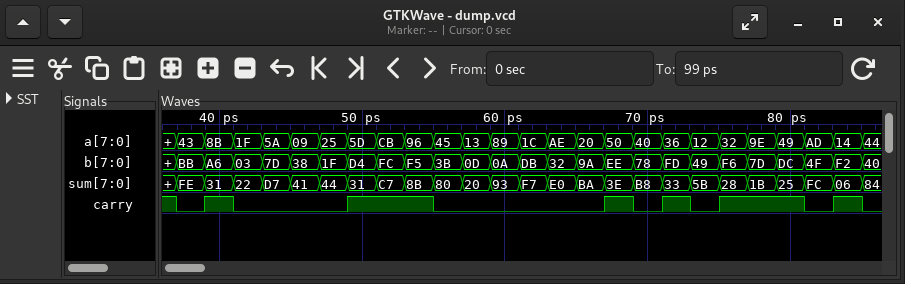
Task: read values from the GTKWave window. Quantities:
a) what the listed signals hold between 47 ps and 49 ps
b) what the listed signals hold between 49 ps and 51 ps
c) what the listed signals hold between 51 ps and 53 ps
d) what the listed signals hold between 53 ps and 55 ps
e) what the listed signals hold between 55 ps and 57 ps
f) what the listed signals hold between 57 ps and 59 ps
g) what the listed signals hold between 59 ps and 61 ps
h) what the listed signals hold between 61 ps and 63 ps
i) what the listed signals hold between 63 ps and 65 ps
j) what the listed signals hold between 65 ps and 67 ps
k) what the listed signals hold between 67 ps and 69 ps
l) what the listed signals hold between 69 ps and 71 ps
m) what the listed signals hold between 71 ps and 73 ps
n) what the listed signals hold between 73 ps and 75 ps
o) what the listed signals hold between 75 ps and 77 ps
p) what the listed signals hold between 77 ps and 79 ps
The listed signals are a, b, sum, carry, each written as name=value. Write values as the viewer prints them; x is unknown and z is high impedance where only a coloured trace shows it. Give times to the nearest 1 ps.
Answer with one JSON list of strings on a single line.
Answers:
["a=25, b=1F, sum=44, carry=0", "a=5D, b=D4, sum=31, carry=1", "a=CB, b=FC, sum=C7, carry=1", "a=96, b=F5, sum=8B, carry=1", "a=45, b=3B, sum=80, carry=0", "a=13, b=0D, sum=20, carry=0", "a=89, b=0A, sum=93, carry=0", "a=1C, b=DB, sum=F7, carry=0", "a=AE, b=32, sum=E0, carry=0", "a=20, b=9A, sum=BA, carry=0", "a=50, b=EE, sum=3E, carry=1", "a=40, b=78, sum=B8, carry=0", "a=36, b=FD, sum=33, carry=1", "a=12, b=49, sum=5B, carry=0", "a=32, b=F6, sum=28, carry=1", "a=9E, b=7D, sum=1B, carry=1"]
